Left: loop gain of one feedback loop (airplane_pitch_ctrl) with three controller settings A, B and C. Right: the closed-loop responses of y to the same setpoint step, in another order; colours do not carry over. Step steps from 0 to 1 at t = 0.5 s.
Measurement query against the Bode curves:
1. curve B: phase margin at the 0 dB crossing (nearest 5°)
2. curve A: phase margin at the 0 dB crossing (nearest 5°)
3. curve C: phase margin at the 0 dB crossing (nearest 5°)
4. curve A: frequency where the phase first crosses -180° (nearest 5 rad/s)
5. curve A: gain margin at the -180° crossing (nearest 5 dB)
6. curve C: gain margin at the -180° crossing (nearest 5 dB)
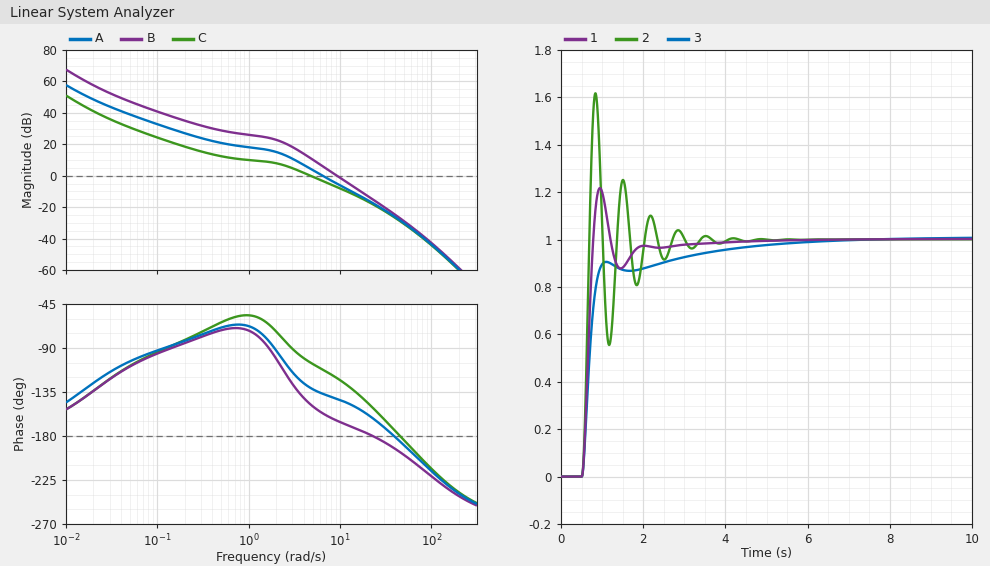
15°
45°
75°
40 rad/s
25 dB
30 dB
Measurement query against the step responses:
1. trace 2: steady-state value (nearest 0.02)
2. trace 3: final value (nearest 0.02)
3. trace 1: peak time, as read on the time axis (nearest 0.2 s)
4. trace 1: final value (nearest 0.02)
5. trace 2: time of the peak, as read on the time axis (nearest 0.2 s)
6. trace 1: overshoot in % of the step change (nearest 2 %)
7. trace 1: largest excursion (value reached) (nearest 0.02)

1.00
1.00
1.0 s
1.00
0.8 s
22 %
1.22
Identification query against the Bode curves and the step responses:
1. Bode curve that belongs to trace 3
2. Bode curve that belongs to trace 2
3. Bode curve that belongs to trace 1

C
B
A
